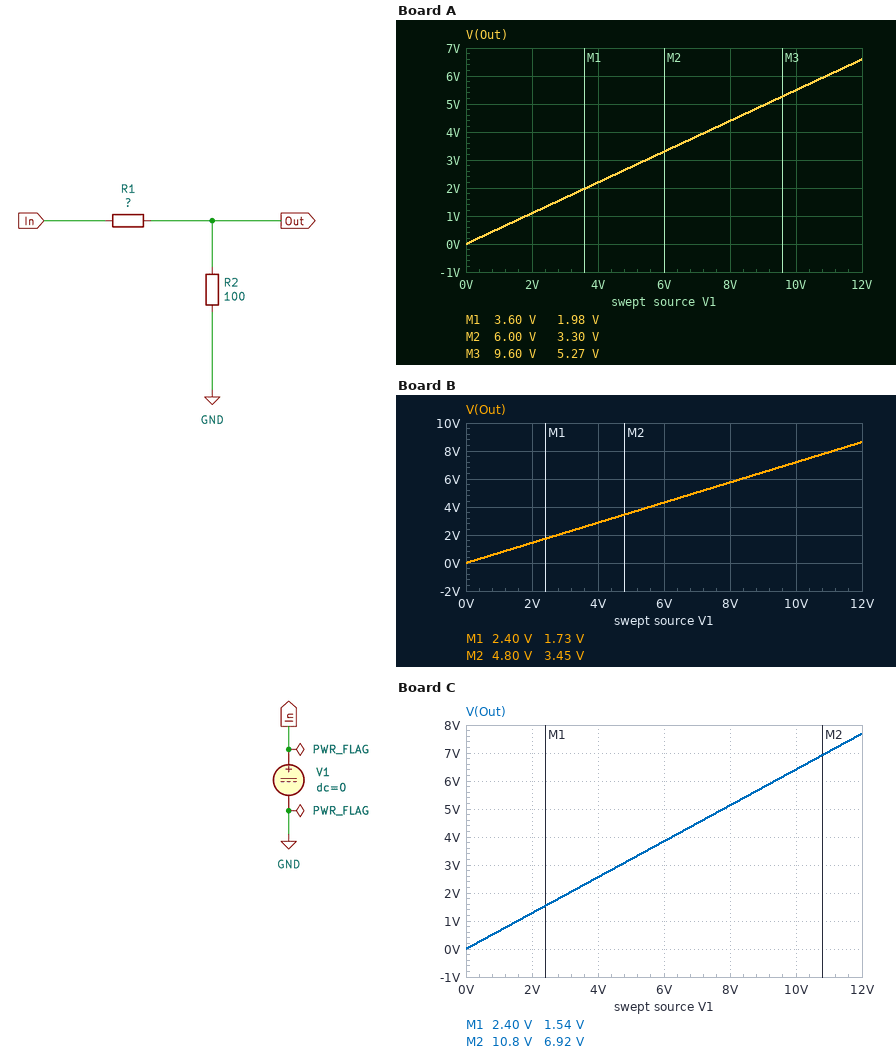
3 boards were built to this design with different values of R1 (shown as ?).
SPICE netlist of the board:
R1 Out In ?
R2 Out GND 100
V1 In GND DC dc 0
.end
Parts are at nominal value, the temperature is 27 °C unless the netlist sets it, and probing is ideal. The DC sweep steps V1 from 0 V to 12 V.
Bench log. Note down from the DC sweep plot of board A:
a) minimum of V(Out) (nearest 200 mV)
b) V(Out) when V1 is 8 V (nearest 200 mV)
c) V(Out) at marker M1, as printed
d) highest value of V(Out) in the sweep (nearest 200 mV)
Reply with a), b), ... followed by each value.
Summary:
a) 0 V
b) 4.4 V
c) 1.98 V
d) 6.6 V
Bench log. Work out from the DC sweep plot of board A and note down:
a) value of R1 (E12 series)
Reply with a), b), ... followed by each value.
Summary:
a) 82 Ω
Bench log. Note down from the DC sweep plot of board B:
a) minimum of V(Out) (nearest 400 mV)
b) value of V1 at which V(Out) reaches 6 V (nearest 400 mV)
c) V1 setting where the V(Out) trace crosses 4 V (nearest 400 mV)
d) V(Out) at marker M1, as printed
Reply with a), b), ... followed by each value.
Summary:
a) 0 V
b) 8.4 V
c) 5.6 V
d) 1.73 V
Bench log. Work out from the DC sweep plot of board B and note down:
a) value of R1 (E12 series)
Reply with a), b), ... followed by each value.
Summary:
a) 39 Ω
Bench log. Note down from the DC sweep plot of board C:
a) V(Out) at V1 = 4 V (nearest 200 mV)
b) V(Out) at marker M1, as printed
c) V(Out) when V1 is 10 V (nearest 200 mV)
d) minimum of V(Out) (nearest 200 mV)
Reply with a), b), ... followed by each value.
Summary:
a) 2.6 V
b) 1.54 V
c) 6.4 V
d) 0 V
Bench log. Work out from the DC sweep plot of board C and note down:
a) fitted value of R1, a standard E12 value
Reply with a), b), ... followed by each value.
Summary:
a) 56 Ω
